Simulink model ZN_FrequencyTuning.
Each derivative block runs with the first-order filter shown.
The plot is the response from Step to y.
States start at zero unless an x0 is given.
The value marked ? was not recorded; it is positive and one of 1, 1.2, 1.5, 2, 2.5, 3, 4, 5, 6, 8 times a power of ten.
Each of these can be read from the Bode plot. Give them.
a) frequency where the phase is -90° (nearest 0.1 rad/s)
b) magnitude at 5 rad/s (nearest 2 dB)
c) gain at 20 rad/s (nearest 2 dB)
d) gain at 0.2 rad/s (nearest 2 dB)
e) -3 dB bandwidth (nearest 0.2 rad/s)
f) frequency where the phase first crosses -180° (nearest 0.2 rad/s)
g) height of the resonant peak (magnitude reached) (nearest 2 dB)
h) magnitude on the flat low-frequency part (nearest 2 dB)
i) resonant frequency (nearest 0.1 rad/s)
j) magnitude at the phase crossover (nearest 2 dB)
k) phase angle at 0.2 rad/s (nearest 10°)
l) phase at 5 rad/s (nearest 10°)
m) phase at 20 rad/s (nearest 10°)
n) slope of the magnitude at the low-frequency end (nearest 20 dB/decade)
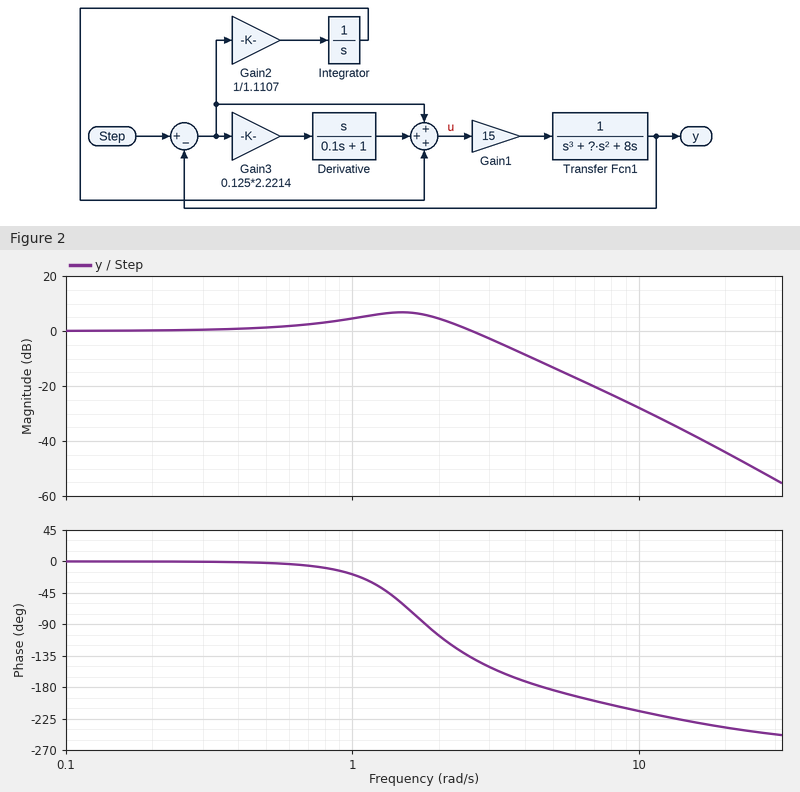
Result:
1.8 rad/s
-14 dB
-44 dB
0 dB
3.0 rad/s
4.6 rad/s
6 dB
0 dB
1.5 rad/s
-12 dB
0°
-180°
-240°
0 dB/decade
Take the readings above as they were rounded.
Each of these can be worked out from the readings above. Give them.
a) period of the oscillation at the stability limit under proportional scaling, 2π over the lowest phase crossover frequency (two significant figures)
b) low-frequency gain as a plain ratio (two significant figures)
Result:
1.4 s
1.0
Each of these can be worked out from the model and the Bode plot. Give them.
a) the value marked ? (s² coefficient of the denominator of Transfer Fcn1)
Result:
5
